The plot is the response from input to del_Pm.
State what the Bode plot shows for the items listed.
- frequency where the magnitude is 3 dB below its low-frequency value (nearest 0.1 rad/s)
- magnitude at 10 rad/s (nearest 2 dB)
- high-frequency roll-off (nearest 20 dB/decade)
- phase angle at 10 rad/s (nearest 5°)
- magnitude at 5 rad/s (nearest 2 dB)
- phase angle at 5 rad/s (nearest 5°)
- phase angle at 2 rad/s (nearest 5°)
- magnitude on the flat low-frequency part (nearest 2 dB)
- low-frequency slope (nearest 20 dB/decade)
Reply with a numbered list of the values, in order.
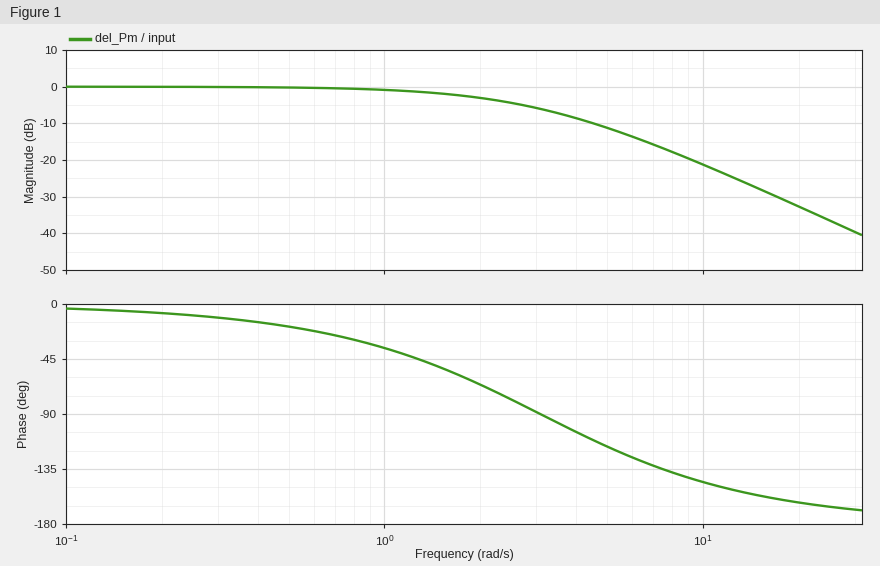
1. 2.0 rad/s
2. -22 dB
3. -40 dB/decade
4. -145°
5. -12 dB
6. -115°
7. -65°
8. 0 dB
9. 0 dB/decade
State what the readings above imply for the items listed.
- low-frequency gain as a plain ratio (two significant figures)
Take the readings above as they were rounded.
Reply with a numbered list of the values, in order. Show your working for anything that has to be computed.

1. 10^(0 / 20) = 1.0
